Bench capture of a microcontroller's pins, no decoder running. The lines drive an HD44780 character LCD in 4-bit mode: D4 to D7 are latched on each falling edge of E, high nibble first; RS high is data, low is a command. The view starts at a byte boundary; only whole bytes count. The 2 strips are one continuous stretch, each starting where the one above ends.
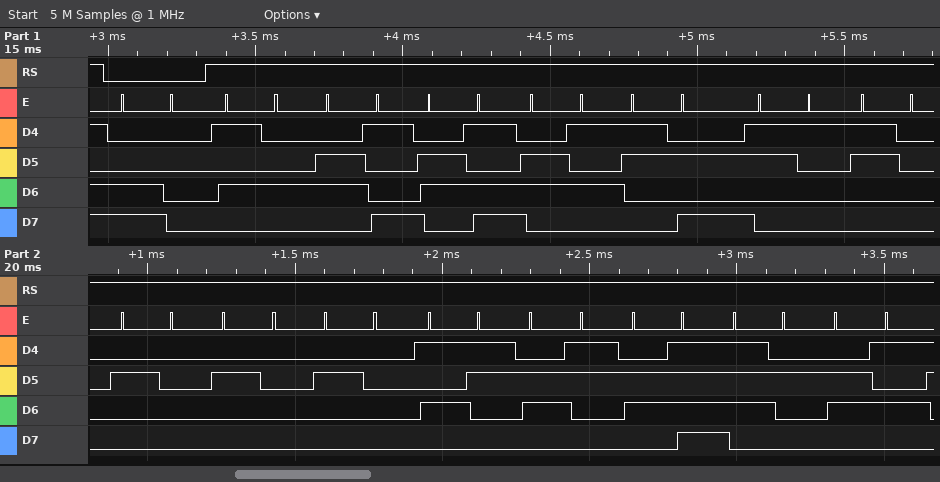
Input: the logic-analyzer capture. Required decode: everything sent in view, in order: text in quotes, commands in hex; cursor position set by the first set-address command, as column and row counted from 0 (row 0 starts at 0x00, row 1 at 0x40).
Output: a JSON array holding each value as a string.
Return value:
["0xC0 \"Time:10   Score\"", "column 0, row 1"]
